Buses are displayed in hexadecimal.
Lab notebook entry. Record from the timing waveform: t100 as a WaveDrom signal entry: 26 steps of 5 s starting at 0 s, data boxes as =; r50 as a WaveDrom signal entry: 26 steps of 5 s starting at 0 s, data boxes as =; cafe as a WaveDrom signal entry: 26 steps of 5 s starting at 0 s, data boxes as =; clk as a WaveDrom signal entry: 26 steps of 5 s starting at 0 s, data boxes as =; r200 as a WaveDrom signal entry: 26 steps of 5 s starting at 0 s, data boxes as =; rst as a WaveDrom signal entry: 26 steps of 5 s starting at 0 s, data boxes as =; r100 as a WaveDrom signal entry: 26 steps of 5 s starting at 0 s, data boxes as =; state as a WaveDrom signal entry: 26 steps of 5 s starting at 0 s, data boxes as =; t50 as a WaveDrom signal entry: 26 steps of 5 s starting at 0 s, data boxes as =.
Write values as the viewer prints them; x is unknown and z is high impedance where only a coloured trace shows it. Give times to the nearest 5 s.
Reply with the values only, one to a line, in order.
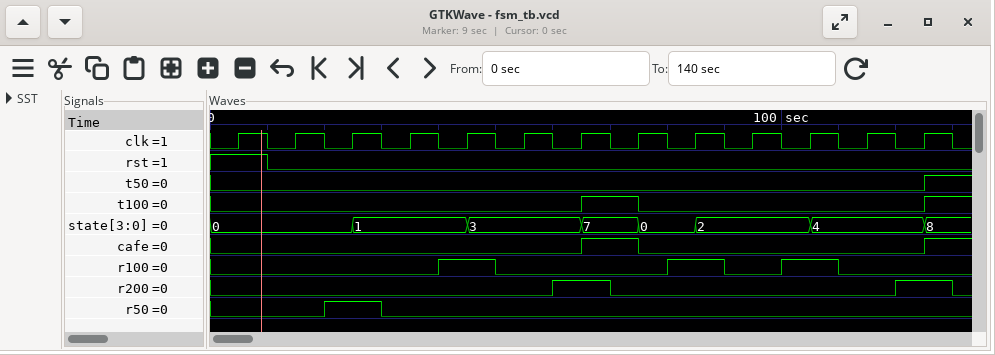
{name: 't100', wave: '0............1.0.........1'}
{name: 'r50', wave: '0...1.0...................'}
{name: 'cafe', wave: '0............1.0.........1'}
{name: 'clk', wave: '01010101010101010101010101'}
{name: 'r200', wave: '0...........1.0.........1.'}
{name: 'rst', wave: '1.0.......................'}
{name: 'r100', wave: '0.......1.0.....1.0.1.0...'}
{name: 'state', wave: '=....=...=...=.=.=...=...=', data: '0 1 3 7 0 2 4 8'}
{name: 't50', wave: '0........................1'}
